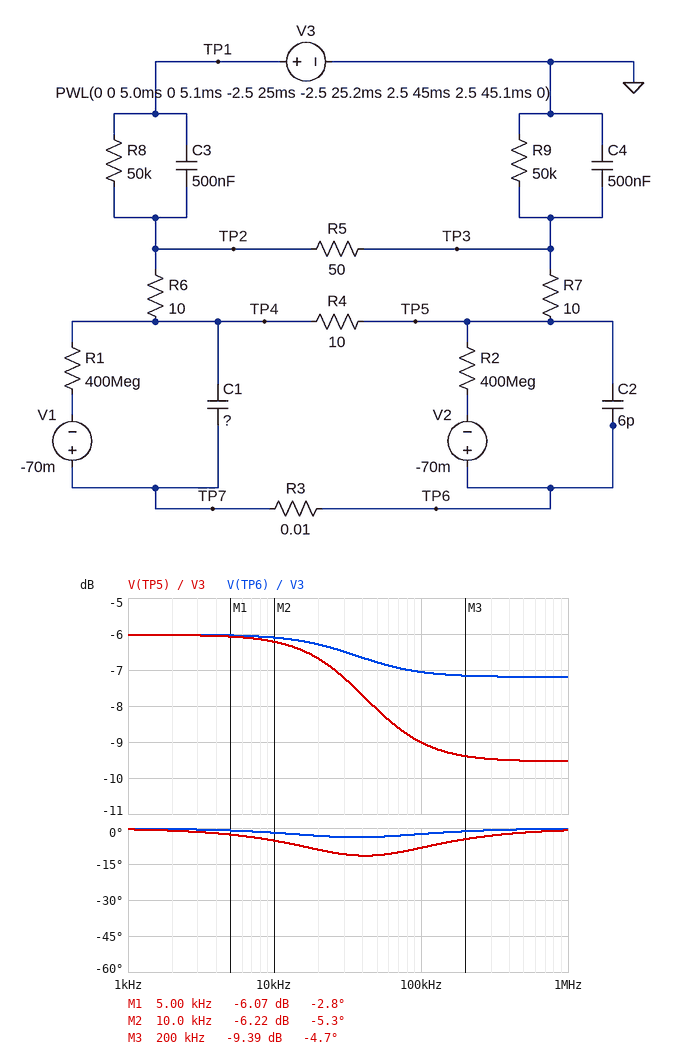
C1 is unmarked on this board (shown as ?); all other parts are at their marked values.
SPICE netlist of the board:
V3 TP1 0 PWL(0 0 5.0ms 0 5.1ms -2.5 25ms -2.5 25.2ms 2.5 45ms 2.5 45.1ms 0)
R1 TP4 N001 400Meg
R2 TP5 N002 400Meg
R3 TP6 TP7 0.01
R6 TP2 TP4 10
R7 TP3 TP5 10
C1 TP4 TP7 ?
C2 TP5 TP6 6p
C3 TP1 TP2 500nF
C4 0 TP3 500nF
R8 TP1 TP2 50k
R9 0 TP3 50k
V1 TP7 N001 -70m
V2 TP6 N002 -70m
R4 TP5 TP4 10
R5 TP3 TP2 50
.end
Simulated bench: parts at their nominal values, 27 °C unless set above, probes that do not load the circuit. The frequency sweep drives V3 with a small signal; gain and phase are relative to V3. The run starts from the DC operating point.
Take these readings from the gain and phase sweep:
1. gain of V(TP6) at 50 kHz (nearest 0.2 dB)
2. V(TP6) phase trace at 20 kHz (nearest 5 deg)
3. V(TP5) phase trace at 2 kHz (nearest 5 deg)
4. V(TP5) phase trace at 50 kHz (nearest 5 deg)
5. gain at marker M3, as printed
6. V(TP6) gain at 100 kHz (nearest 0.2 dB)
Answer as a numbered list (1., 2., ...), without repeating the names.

1. -6.8 dB
2. -5 deg
3. 0 deg
4. -10 deg
5. -9.39 dB
6. -7.0 dB
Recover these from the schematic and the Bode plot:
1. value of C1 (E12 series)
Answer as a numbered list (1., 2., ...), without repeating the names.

1. 2.7 pF
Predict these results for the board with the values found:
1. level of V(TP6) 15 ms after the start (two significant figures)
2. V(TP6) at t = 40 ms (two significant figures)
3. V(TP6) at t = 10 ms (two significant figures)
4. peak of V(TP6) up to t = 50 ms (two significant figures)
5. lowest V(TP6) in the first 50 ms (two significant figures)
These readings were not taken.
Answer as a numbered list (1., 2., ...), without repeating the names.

1. -1.3 V
2. 1.2 V
3. -1.3 V
4. 1.2 V
5. -1.3 V
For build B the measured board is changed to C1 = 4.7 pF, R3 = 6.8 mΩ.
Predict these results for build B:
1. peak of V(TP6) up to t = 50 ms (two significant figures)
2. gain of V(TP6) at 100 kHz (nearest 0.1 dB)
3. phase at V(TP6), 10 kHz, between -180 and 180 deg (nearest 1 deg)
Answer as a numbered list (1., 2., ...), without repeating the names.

1. 1.2 V
2. -6.3 dB
3. -1 deg
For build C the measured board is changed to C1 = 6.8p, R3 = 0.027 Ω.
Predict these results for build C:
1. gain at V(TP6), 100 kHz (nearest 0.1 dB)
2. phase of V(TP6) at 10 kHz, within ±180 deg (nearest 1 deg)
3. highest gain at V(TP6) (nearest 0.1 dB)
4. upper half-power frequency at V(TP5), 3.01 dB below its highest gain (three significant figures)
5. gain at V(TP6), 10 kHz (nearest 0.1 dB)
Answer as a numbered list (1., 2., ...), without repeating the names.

1. -5.9 dB
2. 0 deg
3. -5.8 dB
4. 102 kHz
5. -6.0 dB
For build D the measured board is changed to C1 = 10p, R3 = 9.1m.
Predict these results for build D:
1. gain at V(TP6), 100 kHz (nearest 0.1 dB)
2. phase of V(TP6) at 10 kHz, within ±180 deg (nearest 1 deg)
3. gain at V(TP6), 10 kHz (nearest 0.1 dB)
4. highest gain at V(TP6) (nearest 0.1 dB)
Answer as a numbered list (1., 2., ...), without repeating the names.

1. -5.4 dB
2. 1 deg
3. -6.0 dB
4. -5.3 dB
